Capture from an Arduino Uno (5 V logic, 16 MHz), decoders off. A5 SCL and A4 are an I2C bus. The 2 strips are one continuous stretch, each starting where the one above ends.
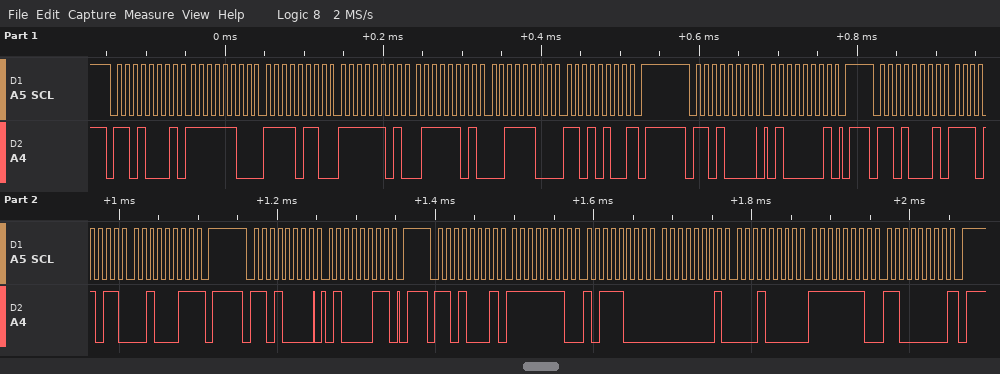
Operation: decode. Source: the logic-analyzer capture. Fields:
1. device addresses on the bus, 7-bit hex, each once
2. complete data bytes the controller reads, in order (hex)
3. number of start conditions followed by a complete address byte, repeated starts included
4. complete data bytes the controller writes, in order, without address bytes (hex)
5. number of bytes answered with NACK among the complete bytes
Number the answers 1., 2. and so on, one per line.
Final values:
1. 0x68
2. FC F6 FD 7D 3C D4 EB 23 FE B8 01 10 FE C0
3. 5
4. 41 43
5. 3
